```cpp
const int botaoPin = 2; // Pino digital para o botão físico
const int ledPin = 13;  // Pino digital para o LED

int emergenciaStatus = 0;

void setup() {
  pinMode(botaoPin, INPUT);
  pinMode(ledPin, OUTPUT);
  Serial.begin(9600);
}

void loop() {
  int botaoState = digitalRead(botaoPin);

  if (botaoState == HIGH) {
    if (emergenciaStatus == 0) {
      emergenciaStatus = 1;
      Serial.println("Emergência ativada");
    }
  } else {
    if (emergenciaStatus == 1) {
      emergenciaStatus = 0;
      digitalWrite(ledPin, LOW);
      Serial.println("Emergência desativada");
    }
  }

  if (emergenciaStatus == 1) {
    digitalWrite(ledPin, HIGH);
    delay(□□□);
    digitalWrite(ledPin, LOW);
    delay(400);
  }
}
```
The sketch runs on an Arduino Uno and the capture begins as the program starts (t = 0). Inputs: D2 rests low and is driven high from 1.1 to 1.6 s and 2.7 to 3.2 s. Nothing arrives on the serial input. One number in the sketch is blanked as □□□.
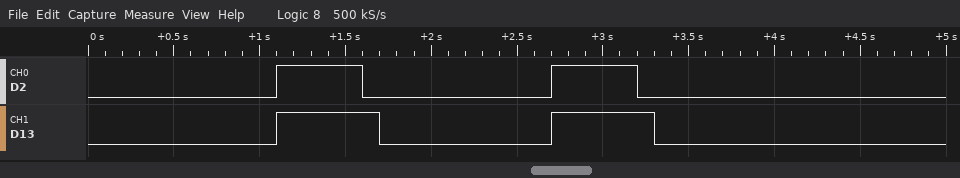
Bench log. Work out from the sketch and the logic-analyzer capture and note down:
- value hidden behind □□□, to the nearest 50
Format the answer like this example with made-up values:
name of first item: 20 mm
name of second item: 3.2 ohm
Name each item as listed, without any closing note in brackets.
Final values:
value hidden behind □□□, to the nearest 50: 600
